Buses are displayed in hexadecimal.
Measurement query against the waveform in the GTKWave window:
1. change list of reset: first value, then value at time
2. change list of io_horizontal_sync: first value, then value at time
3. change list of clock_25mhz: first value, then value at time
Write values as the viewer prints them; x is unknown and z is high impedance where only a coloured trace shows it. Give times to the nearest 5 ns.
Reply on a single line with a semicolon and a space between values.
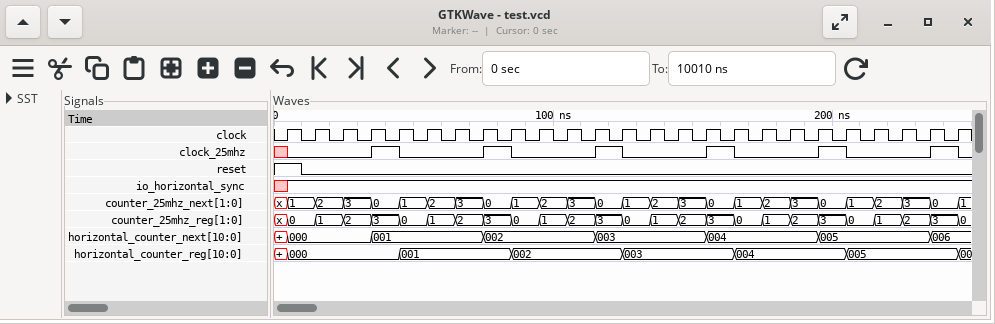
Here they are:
1, 0 at 10 ns; x, 1 at 5 ns; x, 0 at 5 ns, 1 at 35 ns, 0 at 45 ns, 1 at 75 ns, 0 at 85 ns, 1 at 115 ns, 0 at 125 ns, 1 at 155 ns, 0 at 165 ns, 1 at 195 ns, 0 at 205 ns, 1 at 235 ns, 0 at 245 ns
